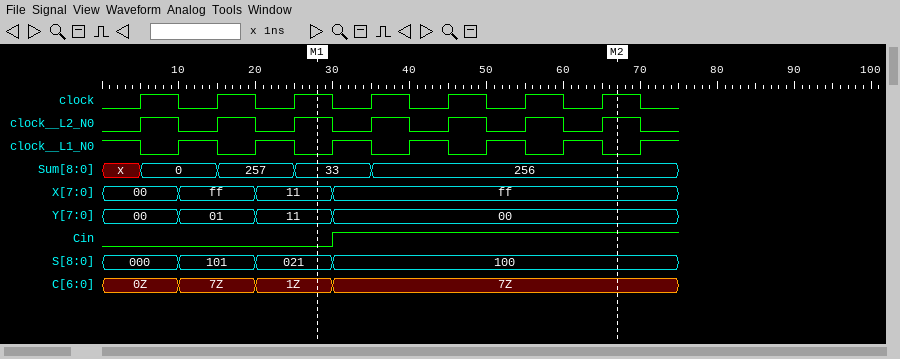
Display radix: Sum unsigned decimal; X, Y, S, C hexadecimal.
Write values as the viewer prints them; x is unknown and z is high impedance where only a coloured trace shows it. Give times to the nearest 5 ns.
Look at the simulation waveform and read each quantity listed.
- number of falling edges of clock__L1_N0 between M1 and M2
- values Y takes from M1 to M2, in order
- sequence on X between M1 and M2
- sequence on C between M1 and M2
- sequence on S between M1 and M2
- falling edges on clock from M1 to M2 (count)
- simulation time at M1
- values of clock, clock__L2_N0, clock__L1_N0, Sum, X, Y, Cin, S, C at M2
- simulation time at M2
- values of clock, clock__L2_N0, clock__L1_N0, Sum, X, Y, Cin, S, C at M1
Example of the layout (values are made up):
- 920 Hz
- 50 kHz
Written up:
- 4
- 11, 00
- 11, ff
- 1Z, 7Z
- 021, 100
- 4
- 30 ns
- clock=1, clock__L2_N0=1, clock__L1_N0=0, Sum=256, X=ff, Y=00, Cin=1, S=100, C=7Z
- 65 ns
- clock=1, clock__L2_N0=1, clock__L1_N0=0, Sum=33, X=11, Y=11, Cin=0, S=021, C=1Z
